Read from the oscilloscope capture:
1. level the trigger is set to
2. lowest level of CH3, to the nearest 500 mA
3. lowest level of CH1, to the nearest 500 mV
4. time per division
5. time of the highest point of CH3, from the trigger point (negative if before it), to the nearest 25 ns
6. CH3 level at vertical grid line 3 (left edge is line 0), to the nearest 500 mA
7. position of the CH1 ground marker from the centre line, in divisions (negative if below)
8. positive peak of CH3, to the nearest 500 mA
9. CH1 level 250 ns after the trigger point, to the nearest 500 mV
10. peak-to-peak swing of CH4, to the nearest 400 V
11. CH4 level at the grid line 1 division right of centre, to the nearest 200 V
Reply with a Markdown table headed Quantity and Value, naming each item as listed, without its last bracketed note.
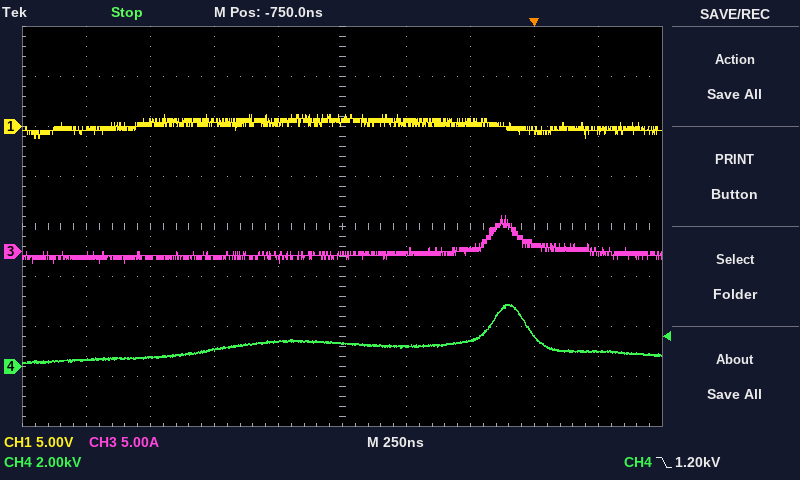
| Quantity | Value |
|---|---|
| level the trigger is set to | 1.20 kV |
| lowest level of CH3, to the nearest 500 mA | -1.0 A |
| lowest level of CH1, to the nearest 500 mV | -1.0 V |
| time per division | 250 ns |
| time of the highest point of CH3, from the trigger point (negative if before it), to the nearest 25 ns | -125 ns |
| CH3 level at vertical grid line 3 (left edge is line 0), to the nearest 500 mA | -500 mA |
| position of the CH1 ground marker from the centre line, in divisions | +2.0 div |
| positive peak of CH3, to the nearest 500 mA | 3.5 A |
| CH1 level 250 ns after the trigger point, to the nearest 500 mV | -500 mV |
| peak-to-peak swing of CH4, to the nearest 400 V | 2.4 kV |
| CH4 level at the grid line 1 division right of centre, to the nearest 200 V | 800 V |
